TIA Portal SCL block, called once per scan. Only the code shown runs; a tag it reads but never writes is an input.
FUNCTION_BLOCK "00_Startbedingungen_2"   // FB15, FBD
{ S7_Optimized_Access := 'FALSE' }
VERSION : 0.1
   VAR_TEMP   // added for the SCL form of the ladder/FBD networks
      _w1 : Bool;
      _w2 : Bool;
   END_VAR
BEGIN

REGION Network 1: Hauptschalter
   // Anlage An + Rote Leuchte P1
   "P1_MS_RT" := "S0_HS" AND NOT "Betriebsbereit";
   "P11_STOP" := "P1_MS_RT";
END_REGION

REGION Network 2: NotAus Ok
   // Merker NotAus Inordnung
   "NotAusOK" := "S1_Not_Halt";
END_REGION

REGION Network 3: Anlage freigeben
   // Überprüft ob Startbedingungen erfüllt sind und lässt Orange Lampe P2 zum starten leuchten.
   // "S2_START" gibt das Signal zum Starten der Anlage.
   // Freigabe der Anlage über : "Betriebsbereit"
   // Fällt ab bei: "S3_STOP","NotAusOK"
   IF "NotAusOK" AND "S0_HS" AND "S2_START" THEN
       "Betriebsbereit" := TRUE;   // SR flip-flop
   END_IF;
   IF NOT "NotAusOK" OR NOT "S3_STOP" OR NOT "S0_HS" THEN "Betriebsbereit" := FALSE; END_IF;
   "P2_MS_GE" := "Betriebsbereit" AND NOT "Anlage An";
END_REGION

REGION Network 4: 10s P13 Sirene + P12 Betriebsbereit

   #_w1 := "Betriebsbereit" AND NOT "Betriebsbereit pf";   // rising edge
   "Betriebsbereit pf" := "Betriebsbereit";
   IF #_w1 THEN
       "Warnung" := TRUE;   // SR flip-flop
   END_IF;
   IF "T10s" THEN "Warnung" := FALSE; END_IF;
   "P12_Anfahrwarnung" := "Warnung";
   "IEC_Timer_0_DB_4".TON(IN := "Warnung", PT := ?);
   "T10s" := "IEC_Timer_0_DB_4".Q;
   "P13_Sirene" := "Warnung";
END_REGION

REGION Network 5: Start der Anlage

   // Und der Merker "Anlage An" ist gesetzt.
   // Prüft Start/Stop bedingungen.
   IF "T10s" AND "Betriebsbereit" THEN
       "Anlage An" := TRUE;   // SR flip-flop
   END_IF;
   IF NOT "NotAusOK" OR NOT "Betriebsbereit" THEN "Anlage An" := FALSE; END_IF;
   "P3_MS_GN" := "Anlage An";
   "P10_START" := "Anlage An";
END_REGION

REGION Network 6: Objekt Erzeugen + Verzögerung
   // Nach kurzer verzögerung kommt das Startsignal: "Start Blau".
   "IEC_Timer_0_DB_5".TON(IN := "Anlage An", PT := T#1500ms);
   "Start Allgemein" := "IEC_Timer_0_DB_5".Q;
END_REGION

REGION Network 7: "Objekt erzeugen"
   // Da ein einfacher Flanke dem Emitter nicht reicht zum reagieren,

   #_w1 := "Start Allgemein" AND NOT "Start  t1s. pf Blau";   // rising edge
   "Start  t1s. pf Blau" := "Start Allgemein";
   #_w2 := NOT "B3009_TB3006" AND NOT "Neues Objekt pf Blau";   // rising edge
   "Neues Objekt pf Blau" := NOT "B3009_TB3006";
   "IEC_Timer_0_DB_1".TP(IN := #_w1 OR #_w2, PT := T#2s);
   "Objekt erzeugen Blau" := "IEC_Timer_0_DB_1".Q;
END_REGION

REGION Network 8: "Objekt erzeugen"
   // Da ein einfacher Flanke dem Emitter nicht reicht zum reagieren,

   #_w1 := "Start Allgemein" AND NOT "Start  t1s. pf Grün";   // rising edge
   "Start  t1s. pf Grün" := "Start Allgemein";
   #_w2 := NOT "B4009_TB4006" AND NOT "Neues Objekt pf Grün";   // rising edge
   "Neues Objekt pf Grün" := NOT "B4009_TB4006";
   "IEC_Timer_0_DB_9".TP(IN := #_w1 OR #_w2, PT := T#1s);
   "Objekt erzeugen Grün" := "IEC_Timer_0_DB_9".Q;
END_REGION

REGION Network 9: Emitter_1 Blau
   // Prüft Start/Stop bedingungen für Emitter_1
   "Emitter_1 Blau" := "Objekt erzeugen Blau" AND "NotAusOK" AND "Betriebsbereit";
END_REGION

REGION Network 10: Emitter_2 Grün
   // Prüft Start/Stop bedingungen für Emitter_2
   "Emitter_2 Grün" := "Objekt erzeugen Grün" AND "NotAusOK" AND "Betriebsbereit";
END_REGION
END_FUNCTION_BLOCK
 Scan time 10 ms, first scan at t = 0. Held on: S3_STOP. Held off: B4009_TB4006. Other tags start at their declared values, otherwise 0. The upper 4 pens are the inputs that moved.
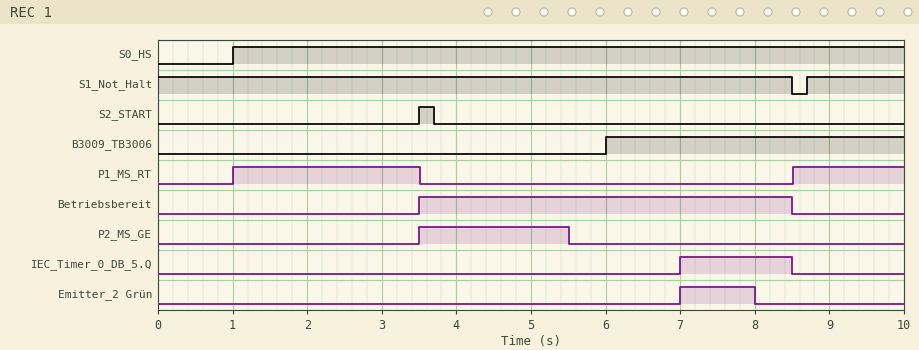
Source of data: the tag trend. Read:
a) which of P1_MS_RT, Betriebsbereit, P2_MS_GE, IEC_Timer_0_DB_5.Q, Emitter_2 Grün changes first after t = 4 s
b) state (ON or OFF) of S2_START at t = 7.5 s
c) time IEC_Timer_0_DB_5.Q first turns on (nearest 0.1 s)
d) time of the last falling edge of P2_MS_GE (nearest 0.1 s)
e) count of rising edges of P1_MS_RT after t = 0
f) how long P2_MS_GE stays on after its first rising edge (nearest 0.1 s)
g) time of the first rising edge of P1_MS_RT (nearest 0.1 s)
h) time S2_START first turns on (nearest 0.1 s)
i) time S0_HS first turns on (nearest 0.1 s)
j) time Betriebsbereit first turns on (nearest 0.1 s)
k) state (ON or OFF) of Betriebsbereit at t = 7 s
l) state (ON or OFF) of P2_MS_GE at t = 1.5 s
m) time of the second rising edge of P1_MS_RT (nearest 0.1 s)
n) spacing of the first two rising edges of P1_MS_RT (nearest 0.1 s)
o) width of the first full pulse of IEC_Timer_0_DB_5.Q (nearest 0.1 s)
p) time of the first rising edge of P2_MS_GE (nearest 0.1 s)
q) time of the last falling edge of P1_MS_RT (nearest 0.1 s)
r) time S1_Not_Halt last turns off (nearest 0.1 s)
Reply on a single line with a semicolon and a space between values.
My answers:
P2_MS_GE; OFF; 7.0 s; 5.5 s; 2; 2.0 s; 1.0 s; 3.5 s; 1.0 s; 3.5 s; ON; OFF; 8.5 s; 7.5 s; 1.5 s; 3.5 s; 3.5 s; 8.5 s
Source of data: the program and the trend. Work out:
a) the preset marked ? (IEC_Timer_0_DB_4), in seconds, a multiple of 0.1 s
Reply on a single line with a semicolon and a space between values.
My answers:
2.0 s
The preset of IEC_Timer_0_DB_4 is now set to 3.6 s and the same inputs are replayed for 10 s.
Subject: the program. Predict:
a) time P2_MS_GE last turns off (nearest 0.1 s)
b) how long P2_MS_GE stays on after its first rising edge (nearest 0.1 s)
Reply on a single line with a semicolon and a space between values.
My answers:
7.1 s; 3.6 s
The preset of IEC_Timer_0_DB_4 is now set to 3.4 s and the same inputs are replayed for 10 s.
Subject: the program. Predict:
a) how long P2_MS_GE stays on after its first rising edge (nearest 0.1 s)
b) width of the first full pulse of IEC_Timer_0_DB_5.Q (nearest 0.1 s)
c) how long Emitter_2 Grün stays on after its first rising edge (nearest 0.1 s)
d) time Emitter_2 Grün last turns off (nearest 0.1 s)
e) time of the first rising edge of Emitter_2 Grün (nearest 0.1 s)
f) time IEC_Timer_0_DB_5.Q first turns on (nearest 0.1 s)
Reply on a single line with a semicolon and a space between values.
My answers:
3.4 s; 0.1 s; 0.1 s; 8.5 s; 8.4 s; 8.4 s
